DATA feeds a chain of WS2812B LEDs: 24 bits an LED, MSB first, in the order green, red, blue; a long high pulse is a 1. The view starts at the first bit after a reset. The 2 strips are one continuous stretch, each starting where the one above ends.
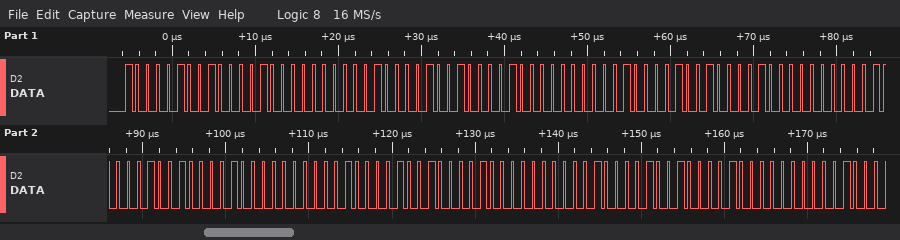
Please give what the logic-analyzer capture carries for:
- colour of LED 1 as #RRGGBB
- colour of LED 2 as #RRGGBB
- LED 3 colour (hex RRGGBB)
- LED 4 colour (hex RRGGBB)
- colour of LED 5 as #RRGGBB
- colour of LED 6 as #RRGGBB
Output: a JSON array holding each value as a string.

["#848400", "#848400", "#848400", "#848400", "#848400", "#848400"]
